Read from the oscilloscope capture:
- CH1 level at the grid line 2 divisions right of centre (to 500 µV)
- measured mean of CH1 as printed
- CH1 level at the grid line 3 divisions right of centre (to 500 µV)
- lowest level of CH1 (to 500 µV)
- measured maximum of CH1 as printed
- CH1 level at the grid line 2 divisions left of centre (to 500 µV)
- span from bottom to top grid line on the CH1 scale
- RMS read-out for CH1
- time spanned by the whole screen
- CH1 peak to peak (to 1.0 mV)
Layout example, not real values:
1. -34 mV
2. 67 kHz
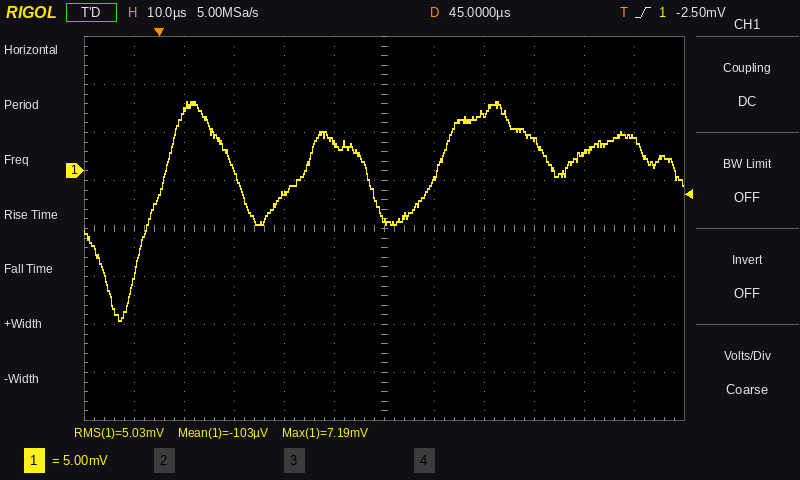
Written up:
1. 6.0 mV
2. -103 µV
3. 3.0 mV
4. -15.5 mV
5. 7.19 mV
6. -2.5 mV
7. 40 mV
8. 5.03 mV
9. 120 µs
10. 23.0 mV
